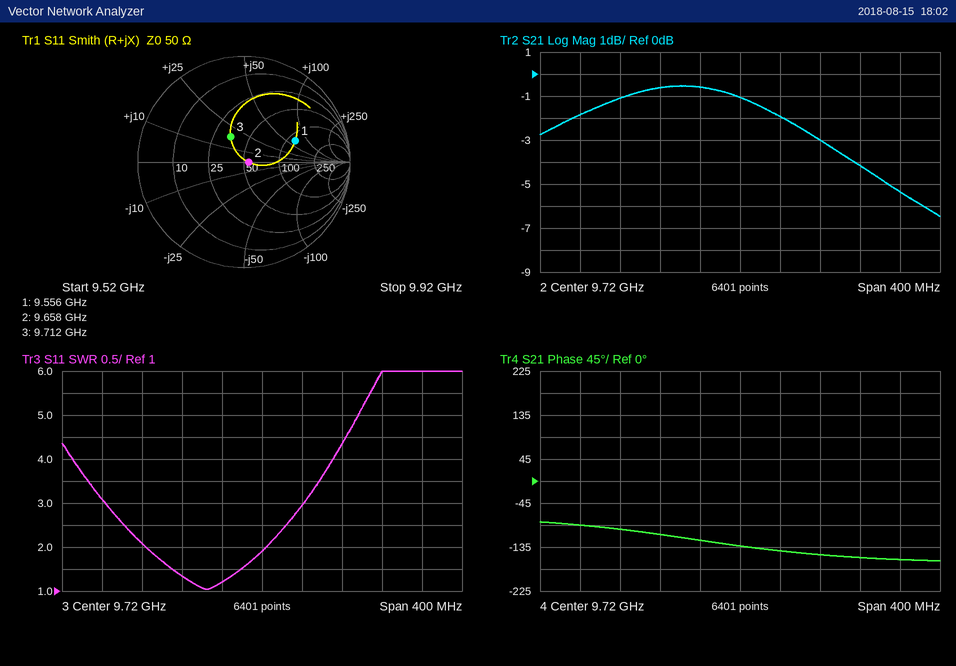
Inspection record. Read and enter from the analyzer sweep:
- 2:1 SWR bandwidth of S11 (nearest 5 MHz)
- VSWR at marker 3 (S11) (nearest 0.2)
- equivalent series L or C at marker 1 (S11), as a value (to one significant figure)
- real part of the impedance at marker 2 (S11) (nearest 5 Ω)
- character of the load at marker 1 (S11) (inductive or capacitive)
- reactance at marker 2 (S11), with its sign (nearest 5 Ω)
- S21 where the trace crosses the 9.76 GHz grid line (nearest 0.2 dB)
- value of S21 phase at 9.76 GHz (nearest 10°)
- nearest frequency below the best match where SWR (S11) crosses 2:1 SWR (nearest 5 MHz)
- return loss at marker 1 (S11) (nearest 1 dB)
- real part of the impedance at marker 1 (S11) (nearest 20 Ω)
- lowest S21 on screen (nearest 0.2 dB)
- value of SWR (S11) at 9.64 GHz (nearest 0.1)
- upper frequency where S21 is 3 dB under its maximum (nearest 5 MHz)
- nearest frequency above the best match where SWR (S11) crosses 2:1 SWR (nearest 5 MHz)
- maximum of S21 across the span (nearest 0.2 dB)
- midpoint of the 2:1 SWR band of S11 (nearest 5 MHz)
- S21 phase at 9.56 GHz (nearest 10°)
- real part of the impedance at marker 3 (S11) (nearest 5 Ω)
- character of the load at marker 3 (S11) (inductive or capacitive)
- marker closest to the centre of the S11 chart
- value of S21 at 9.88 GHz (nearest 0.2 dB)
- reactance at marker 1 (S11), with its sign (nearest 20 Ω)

120 MHz
1.8
1 nH
55 Ω
inductive
0 Ω
-2.0 dB
-140°
9.605 GHz
6 dB
120 Ω
-6.4 dB
1.3
9.820 GHz
9.725 GHz
-0.6 dB
9.665 GHz
-90°
35 Ω
inductive
marker 2
-5.4 dB
+60 Ω
